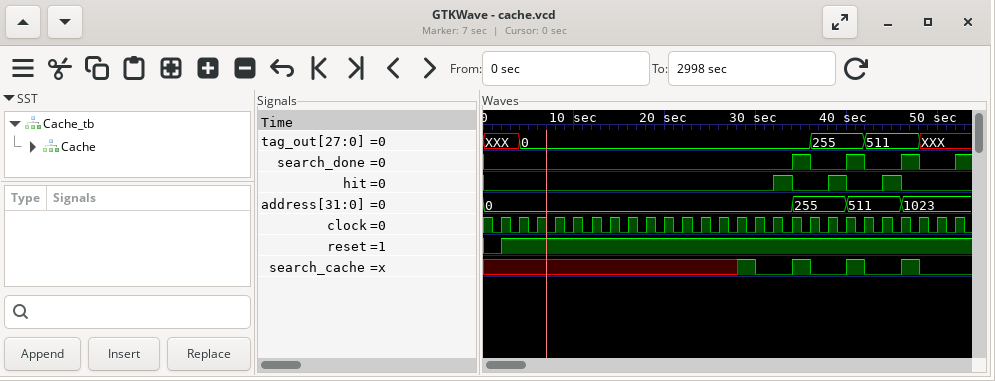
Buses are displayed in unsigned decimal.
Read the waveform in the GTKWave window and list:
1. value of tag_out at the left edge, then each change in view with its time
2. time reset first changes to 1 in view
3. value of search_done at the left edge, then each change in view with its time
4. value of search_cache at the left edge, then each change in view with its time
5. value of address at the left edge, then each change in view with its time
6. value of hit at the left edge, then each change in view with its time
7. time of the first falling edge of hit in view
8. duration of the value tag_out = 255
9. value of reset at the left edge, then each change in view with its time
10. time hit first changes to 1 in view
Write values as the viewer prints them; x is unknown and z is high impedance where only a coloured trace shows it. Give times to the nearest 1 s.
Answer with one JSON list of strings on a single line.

["XXX, 0 at 4 s, 255 at 36 s, 511 at 42 s, XXX at 48 s", "2 s", "0, 1 at 34 s, 0 at 36 s, 1 at 40 s, 0 at 42 s, 1 at 46 s, 0 at 48 s, 1 at 52 s", "x, 1 at 28 s, 0 at 30 s, 1 at 34 s, 0 at 36 s, 1 at 40 s, 0 at 42 s, 1 at 46 s, 0 at 48 s", "0, 255 at 34 s, 511 at 40 s, 1023 at 46 s", "0, 1 at 32 s, 0 at 34 s, 1 at 38 s, 0 at 40 s, 1 at 44 s, 0 at 46 s", "34 s", "6 s", "0, 1 at 2 s", "32 s"]
